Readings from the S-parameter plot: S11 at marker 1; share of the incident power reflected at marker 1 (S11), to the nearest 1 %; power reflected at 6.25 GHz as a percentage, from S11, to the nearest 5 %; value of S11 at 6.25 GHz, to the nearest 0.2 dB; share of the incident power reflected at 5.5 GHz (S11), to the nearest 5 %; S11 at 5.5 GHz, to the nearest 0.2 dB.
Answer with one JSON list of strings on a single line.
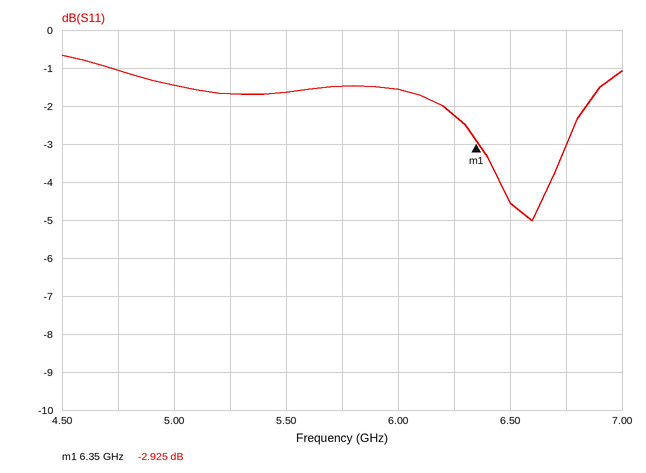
["-2.925 dB", "51 %", "60 %", "-2.2 dB", "70 %", "-1.6 dB"]
